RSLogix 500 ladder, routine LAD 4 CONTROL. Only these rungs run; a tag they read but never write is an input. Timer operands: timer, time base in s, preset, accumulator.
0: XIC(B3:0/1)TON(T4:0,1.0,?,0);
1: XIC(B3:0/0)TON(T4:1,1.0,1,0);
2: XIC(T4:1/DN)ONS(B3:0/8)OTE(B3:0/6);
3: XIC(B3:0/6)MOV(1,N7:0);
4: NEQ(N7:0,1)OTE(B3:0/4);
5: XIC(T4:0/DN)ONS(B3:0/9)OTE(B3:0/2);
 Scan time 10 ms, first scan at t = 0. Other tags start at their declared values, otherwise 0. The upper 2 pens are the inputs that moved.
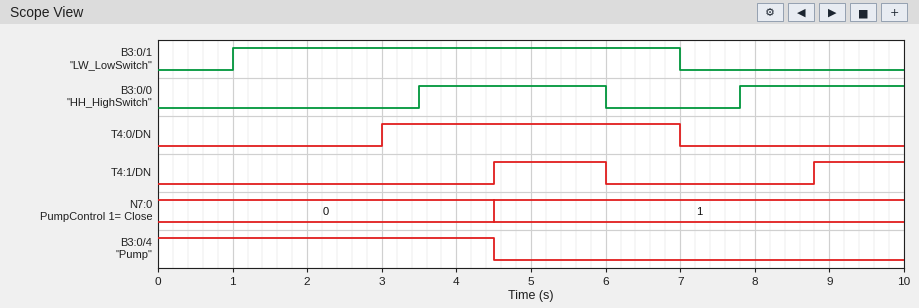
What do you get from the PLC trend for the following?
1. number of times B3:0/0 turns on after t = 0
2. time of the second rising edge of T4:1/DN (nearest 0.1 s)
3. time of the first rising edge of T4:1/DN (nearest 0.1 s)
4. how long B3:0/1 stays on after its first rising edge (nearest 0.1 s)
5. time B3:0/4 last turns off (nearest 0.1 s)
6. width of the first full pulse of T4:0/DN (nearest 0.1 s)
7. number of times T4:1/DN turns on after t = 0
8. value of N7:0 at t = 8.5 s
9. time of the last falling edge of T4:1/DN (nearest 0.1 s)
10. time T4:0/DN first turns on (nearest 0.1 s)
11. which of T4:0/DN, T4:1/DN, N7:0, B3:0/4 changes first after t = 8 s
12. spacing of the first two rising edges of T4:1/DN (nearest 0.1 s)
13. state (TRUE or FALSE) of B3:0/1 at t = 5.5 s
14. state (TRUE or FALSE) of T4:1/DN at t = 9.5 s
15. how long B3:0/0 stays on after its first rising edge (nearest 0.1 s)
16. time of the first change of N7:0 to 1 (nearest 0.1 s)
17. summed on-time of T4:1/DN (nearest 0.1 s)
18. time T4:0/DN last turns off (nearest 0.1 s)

2
8.8 s
4.5 s
6.0 s
4.5 s
4.0 s
2
1
6.0 s
3.0 s
T4:1/DN
4.3 s
TRUE
TRUE
2.5 s
4.5 s
2.7 s
7.0 s
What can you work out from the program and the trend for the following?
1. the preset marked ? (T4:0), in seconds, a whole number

2 s
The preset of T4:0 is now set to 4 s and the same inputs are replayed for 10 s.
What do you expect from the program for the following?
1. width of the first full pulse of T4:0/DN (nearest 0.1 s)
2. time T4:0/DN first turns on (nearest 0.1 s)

2.0 s
5.0 s
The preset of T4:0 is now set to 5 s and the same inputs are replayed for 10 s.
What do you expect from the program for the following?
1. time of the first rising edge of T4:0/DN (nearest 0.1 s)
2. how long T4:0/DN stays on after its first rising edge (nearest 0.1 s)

6.0 s
1.0 s
